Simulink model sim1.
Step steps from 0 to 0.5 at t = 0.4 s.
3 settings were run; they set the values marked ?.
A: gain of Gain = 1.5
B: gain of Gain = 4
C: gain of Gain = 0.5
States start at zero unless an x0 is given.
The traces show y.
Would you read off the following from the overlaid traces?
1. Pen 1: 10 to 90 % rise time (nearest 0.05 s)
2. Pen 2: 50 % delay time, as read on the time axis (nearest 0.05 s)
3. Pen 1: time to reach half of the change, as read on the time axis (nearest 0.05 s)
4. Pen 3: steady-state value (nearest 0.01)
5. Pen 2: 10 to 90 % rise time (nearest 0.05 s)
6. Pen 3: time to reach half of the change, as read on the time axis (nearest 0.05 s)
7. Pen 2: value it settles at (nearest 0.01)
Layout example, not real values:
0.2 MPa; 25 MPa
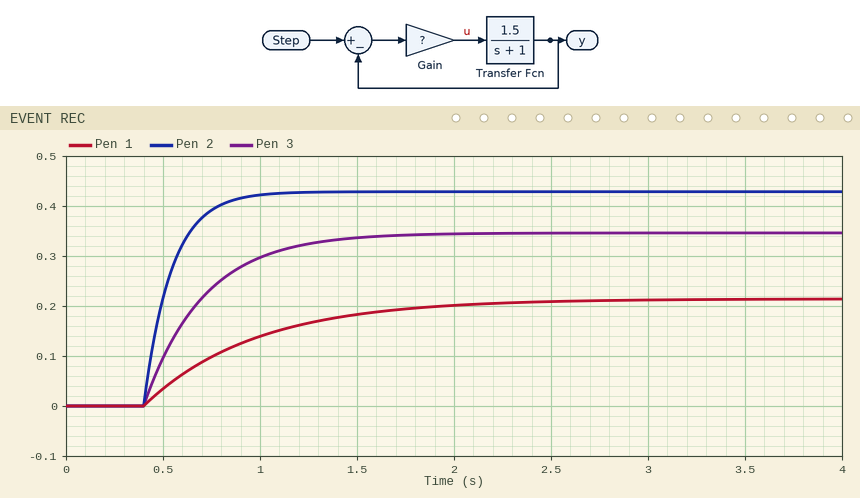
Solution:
1.25 s; 0.50 s; 0.80 s; 0.35; 0.30 s; 0.60 s; 0.43
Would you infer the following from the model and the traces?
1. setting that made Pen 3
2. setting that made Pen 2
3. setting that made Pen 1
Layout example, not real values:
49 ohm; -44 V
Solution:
A; B; C
